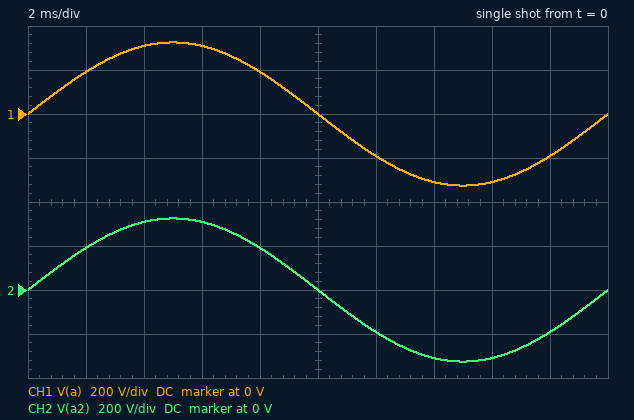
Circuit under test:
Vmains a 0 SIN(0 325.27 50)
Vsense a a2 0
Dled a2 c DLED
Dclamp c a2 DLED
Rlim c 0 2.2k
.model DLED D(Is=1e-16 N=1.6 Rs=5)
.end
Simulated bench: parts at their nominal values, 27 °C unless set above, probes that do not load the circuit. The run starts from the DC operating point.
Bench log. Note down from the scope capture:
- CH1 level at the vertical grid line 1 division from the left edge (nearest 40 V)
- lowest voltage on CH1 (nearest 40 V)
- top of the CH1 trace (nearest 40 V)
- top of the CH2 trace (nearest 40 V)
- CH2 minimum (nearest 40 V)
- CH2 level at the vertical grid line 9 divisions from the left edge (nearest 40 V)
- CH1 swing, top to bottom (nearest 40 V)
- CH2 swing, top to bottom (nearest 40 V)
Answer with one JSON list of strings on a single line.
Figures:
["200 V", "-320 V", "320 V", "320 V", "-320 V", "-200 V", "640 V", "640 V"]
